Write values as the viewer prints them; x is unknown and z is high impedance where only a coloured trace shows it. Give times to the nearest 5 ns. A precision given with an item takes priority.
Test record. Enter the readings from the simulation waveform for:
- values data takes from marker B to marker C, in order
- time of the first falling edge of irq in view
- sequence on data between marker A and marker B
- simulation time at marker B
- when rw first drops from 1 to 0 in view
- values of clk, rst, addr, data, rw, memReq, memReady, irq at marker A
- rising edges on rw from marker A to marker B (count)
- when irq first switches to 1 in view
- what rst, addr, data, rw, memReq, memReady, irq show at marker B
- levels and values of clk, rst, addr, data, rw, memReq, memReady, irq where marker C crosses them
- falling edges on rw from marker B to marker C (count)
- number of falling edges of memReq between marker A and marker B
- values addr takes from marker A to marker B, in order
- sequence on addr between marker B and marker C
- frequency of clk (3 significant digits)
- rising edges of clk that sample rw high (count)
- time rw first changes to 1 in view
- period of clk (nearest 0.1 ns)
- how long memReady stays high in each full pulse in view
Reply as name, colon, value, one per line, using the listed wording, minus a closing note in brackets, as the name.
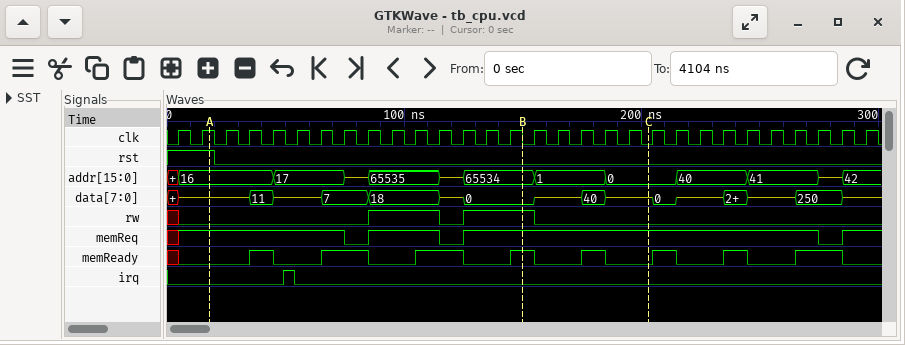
values data takes from marker B to marker C, in order: 0, z, 40, z
time of the first falling edge of irq in view: 55 ns
sequence on data between marker A and marker B: z, 11, z, 7, 18, z, 0
simulation time at marker B: 150 ns
when rw first drops from 1 to 0 in view: 115 ns
values of clk, rst, addr, data, rw, memReq, memReady, irq at marker A: clk=1, rst=1, addr=16, data=z, rw=0, memReq=1, memReady=0, irq=0
rising edges on rw from marker A to marker B: 2
when irq first switches to 1 in view: 50 ns
what rst, addr, data, rw, memReq, memReady, irq show at marker B: rst=0, addr=65534, data=0, rw=1, memReq=1, memReady=1, irq=0
levels and values of clk, rst, addr, data, rw, memReq, memReady, irq where marker C crosses them: clk=0, rst=0, addr=0, data=z, rw=0, memReq=1, memReady=0, irq=0
falling edges on rw from marker B to marker C: 1
number of falling edges of memReq between marker A and marker B: 2
values addr takes from marker A to marker B, in order: 16, 17, z, 65535, z, 65534
sequence on addr between marker B and marker C: 65534, 1, 0
frequency of clk: 100 MHz
rising edges of clk that sample rw high: 6
time rw first changes to 1 in view: 85 ns
period of clk: 10 ns
how long memReady stays high in each full pulse in view: 10 ns, 20 ns, 20 ns, 10 ns, 10 ns, 10 ns, 10 ns, 20 ns
